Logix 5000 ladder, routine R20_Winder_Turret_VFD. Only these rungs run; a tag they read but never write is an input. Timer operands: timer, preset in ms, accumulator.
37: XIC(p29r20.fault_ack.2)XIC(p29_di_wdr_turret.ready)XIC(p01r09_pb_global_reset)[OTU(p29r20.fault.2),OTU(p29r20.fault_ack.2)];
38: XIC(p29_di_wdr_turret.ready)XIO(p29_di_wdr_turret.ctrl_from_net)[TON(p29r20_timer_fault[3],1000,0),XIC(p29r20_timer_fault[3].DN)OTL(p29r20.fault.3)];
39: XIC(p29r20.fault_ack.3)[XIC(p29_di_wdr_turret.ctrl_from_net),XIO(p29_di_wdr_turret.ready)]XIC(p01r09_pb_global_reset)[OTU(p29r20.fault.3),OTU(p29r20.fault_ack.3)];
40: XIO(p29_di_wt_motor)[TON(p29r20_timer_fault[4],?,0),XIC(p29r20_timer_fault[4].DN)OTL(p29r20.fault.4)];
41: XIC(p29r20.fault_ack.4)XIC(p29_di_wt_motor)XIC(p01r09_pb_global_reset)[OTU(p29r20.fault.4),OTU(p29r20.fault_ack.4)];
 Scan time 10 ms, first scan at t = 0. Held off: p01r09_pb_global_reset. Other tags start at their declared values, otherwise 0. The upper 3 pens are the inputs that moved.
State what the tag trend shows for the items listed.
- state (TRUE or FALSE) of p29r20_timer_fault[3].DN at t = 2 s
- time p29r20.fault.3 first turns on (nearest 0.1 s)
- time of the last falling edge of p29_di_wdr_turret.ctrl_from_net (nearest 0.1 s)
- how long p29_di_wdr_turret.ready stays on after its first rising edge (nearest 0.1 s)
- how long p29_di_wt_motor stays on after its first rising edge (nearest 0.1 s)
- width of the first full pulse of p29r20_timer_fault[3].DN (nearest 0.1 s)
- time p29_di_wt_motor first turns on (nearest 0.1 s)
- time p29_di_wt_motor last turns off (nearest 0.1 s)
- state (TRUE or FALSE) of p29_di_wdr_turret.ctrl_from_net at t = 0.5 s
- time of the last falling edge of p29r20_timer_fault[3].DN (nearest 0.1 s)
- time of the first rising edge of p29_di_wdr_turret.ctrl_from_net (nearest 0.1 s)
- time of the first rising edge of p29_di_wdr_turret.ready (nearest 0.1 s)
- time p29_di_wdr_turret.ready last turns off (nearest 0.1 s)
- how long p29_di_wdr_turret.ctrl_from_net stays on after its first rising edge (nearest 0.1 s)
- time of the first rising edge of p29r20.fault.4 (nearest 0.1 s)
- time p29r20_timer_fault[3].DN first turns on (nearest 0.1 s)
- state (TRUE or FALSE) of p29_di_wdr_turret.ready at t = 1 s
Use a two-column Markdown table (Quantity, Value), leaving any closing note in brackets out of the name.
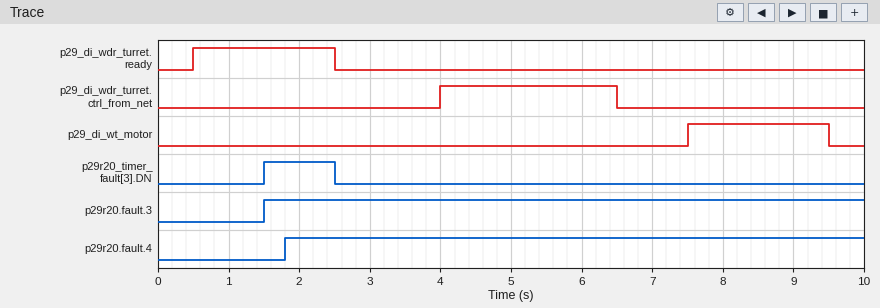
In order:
| Quantity | Value |
|---|---|
| state (TRUE or FALSE) of p29r20_timer_fault[3].DN at t = 2 s | TRUE |
| time p29r20.fault.3 first turns on | 1.5 s |
| time of the last falling edge of p29_di_wdr_turret.ctrl_from_net | 6.5 s |
| how long p29_di_wdr_turret.ready stays on after its first rising edge | 2.0 s |
| how long p29_di_wt_motor stays on after its first rising edge | 2.0 s |
| width of the first full pulse of p29r20_timer_fault[3].DN | 1.0 s |
| time p29_di_wt_motor first turns on | 7.5 s |
| time p29_di_wt_motor last turns off | 9.5 s |
| state (TRUE or FALSE) of p29_di_wdr_turret.ctrl_from_net at t = 0.5 s | FALSE |
| time of the last falling edge of p29r20_timer_fault[3].DN | 2.5 s |
| time of the first rising edge of p29_di_wdr_turret.ctrl_from_net | 4.0 s |
| time of the first rising edge of p29_di_wdr_turret.ready | 0.5 s |
| time p29_di_wdr_turret.ready last turns off | 2.5 s |
| how long p29_di_wdr_turret.ctrl_from_net stays on after its first rising edge | 2.5 s |
| time of the first rising edge of p29r20.fault.4 | 1.8 s |
| time p29r20_timer_fault[3].DN first turns on | 1.5 s |
| state (TRUE or FALSE) of p29_di_wdr_turret.ready at t = 1 s | TRUE |
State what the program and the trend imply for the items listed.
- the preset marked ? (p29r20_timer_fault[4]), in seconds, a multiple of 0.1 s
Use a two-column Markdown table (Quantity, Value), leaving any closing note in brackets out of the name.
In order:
| Quantity | Value |
|---|---|
| the preset marked ? (p29r20_timer_fault[4]), in seconds, a multiple of 0.1 s | 1.8 s |
